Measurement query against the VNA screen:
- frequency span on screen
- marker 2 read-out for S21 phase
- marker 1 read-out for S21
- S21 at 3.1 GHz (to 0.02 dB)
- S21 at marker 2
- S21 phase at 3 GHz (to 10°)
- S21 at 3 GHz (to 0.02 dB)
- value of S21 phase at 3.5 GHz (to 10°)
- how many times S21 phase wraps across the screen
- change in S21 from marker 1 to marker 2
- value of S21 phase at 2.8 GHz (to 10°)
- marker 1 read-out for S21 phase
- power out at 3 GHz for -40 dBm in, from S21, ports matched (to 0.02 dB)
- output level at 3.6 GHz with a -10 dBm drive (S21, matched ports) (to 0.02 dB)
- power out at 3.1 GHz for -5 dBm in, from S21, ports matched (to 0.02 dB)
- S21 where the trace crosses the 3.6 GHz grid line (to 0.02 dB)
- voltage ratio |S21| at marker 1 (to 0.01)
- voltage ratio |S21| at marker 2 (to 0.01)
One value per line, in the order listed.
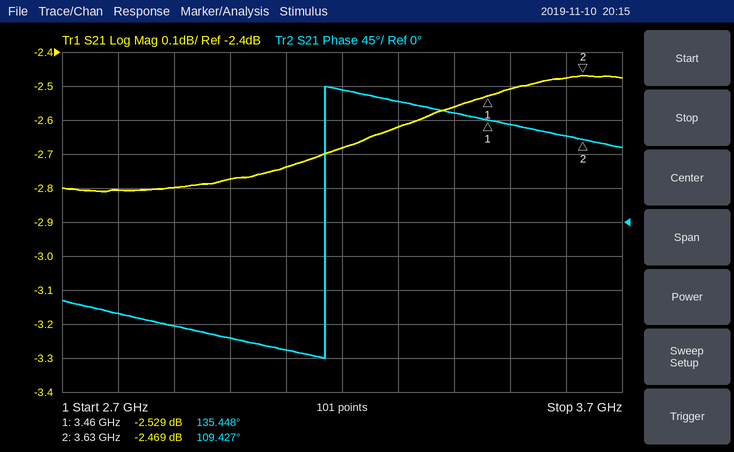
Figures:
1 GHz
109.427°
-2.529 dB
-2.74 dB
-2.469 dB
-150°
-2.78 dB
130°
1
0.060 dB
-120°
135.448°
-42.78 dBm
-12.48 dBm
-7.74 dBm
-2.48 dB
0.75
0.75
